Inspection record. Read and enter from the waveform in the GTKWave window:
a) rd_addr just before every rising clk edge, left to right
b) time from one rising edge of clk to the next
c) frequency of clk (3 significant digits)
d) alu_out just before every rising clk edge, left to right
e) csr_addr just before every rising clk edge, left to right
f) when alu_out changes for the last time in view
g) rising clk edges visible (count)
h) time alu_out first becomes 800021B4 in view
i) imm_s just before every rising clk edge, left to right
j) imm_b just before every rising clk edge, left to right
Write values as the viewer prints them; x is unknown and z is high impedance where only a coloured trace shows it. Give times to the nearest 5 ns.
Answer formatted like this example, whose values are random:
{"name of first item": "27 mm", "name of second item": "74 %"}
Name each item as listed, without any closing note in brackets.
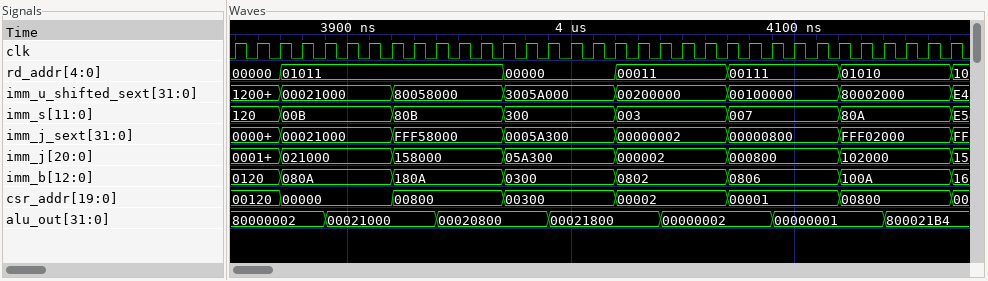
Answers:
{"rd_addr just before every rising clk edge, left to right": "00000, 00000, 00000, 01011, 01011, 01011, 01011, 01011, 01011, 01011, 01011, 01011, 01011, 00000, 00000, 00000, 00000, 00000, 00011, 00011, 00011, 00011, 00011, 00111, 00111, 00111, 00111, 00111, 01010, 01010, 01010, 01010, 01010", "time from one rising edge of clk to the next": "10 ns", "frequency of clk": "100 MHz", "alu_out just before every rising clk edge, left to right": "80000002, 80000002, 80000002, 80000002, 80000002, 00021000, 00021000, 00021000, 00021000, 00021000, 00020800, 00020800, 00020800, 00020800, 00020800, 00021800, 00021800, 00021800, 00021800, 00021800, 00000002, 00000002, 00000002, 00000002, 00000002, 00000001, 00000001, 00000001, 00000001, 00000001, 800021B4, 800021B4, 800021B4", "csr_addr just before every rising clk edge, left to right": "00120, 00120, 00120, 00000, 00000, 00000, 00000, 00000, 00800, 00800, 00800, 00800, 00800, 00300, 00300, 00300, 00300, 00300, 00002, 00002, 00002, 00002, 00002, 00001, 00001, 00001, 00001, 00001, 00800, 00800, 00800, 00800, 00800", "when alu_out changes for the last time in view": "4140 ns", "rising clk edges visible": "33", "time alu_out first becomes 800021B4 in view": "4140 ns", "imm_s just before every rising clk edge, left to right": "120, 120, 120, 00B, 00B, 00B, 00B, 00B, 80B, 80B, 80B, 80B, 80B, 300, 300, 300, 300, 300, 003, 003, 003, 003, 003, 007, 007, 007, 007, 007, 80A, 80A, 80A, 80A, 80A", "imm_b just before every rising clk edge, left to right": "0120, 0120, 0120, 080A, 080A, 080A, 080A, 080A, 180A, 180A, 180A, 180A, 180A, 0300, 0300, 0300, 0300, 0300, 0802, 0802, 0802, 0802, 0802, 0806, 0806, 0806, 0806, 0806, 100A, 100A, 100A, 100A, 100A"}
